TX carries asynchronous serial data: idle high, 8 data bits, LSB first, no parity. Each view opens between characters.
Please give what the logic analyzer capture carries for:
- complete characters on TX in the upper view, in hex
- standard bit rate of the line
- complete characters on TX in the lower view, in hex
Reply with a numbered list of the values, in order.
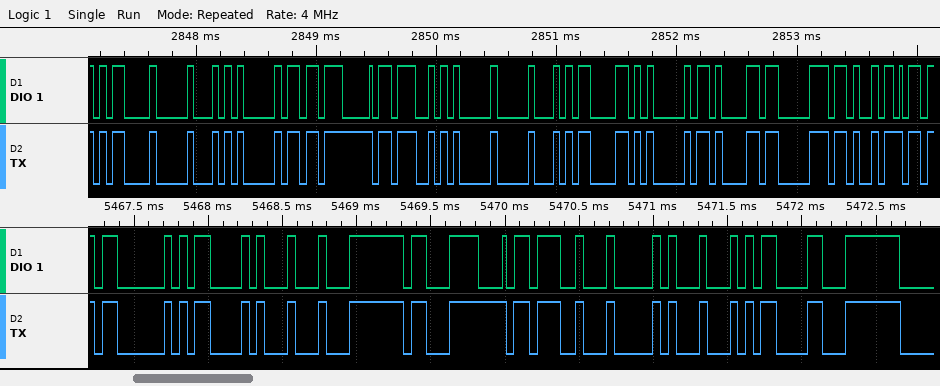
1. 0D, 10, 05, DB, 3B, 05, 10, 0D, 05, 0B, 83, 4B
2. 19200 baud
3. 03, 0D, 11, FC, E3, 3B, 04, 11, 0D, FC
